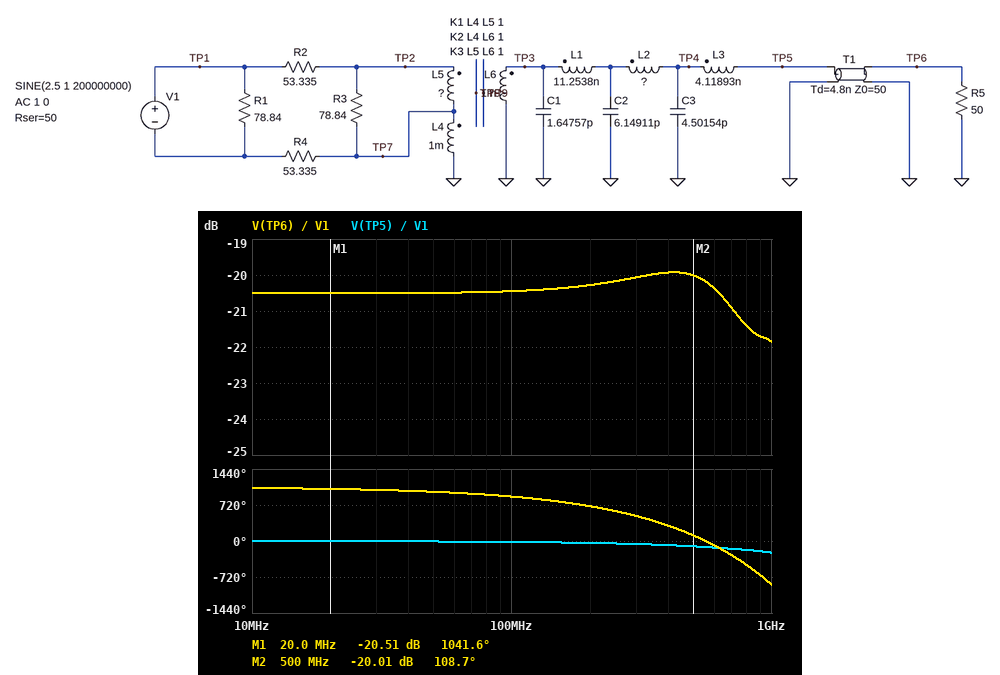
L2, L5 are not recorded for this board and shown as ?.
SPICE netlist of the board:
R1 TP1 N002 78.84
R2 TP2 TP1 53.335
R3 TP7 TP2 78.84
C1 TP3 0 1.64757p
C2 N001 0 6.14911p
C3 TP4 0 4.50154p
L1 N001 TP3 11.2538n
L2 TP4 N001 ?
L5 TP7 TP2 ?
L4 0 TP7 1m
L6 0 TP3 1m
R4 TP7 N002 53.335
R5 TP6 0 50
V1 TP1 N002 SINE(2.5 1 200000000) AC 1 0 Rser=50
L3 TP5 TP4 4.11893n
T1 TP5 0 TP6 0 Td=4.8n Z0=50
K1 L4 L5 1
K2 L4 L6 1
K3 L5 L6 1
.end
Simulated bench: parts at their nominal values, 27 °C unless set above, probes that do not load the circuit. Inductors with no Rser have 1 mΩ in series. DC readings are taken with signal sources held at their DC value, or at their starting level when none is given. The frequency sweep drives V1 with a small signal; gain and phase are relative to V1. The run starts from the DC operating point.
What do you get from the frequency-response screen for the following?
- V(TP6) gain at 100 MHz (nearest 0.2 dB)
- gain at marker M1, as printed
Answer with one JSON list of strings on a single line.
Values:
["-20.4 dB", "-20.51 dB"]
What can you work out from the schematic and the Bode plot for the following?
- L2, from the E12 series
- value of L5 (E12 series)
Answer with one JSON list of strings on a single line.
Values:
["10 nH", "3.3 mH"]
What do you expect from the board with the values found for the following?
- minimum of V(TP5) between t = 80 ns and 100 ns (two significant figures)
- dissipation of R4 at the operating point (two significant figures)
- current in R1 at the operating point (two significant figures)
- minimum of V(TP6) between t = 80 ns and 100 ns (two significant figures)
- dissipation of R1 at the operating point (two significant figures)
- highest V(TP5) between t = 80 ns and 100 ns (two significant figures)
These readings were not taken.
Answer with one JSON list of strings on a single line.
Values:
["-97 mV", "6.6 mW", "15 mA", "-97 mV", "18 mW", "97 mV"]
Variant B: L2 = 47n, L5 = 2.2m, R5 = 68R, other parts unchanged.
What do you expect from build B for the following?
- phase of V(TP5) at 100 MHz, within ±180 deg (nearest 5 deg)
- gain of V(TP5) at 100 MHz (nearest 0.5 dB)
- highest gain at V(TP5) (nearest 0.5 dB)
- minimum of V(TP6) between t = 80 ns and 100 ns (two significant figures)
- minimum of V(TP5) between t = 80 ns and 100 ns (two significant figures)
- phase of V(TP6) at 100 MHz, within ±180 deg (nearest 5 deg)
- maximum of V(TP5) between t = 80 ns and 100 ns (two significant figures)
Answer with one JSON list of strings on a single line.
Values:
["-30 deg", "-19.5 dB", "-19.0 dB", "-100 mV", "-99 mV", "155 deg", "99 mV"]
